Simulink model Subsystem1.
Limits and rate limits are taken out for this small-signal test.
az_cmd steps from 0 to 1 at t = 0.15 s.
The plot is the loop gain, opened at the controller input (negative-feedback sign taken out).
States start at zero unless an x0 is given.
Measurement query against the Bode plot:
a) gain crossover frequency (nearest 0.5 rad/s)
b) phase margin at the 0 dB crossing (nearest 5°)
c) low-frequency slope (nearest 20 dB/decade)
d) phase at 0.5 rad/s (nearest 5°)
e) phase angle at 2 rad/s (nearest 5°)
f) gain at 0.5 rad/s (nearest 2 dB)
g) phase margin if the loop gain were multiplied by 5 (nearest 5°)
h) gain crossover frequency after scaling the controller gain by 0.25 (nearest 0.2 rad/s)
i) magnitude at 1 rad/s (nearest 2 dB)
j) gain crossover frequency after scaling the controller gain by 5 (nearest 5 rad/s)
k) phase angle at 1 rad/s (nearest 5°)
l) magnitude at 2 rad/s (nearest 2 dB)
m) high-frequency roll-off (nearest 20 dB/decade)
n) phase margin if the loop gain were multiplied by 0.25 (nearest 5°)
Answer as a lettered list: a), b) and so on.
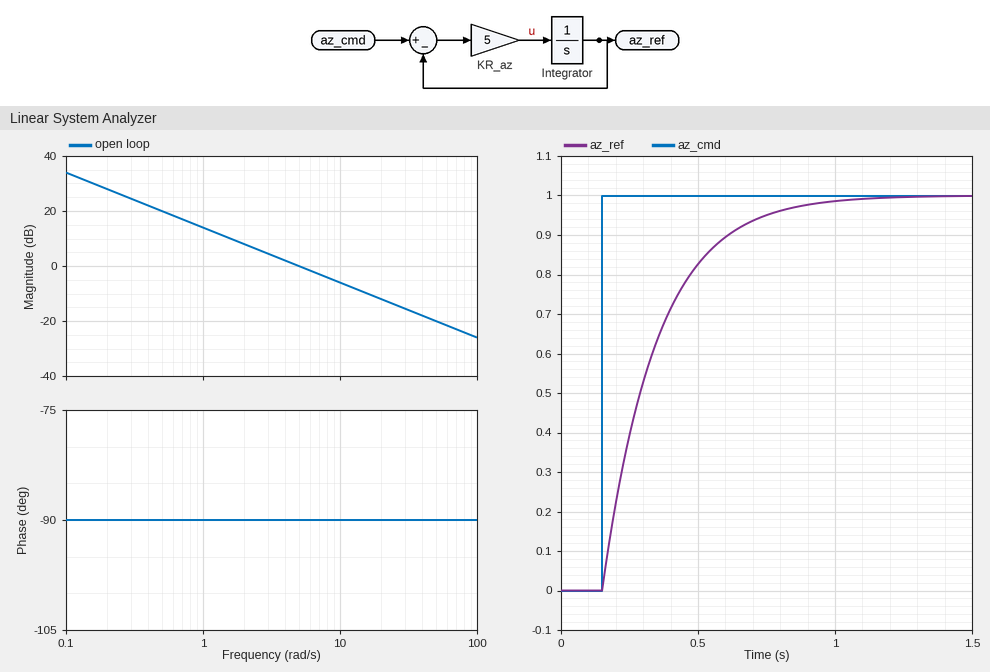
a) 5.0 rad/s
b) 90°
c) -20 dB/decade
d) -90°
e) -90°
f) 20 dB
g) 90°
h) 1.2 rad/s
i) 14 dB
j) 25 rad/s
k) -90°
l) 8 dB
m) -20 dB/decade
n) 90°
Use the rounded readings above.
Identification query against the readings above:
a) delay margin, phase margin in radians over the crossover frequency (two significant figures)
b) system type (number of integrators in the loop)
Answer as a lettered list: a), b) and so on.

a) 0.31 s
b) 1
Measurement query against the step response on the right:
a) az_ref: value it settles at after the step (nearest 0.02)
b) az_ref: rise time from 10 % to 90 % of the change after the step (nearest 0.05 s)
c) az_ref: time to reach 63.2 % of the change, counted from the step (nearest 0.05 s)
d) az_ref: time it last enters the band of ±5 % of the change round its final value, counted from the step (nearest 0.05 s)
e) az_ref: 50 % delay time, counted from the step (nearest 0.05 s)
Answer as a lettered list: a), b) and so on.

a) 1.00
b) 0.45 s
c) 0.20 s
d) 0.60 s
e) 0.15 s
